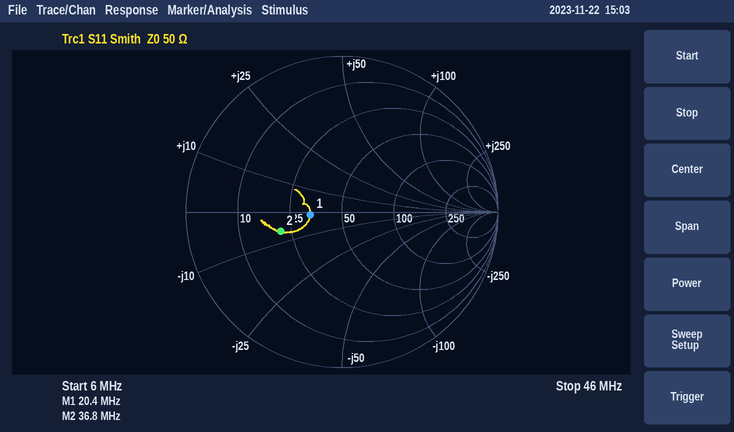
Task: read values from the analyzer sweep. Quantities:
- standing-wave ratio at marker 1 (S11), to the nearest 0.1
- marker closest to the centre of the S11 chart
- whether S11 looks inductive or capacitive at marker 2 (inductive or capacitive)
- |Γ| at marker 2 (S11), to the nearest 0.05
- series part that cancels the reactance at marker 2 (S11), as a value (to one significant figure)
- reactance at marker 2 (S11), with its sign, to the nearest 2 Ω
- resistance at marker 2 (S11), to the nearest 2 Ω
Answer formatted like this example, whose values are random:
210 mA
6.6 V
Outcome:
1.5
marker 1
capacitive
0.40
30 nH
-6 Ω
22 Ω
